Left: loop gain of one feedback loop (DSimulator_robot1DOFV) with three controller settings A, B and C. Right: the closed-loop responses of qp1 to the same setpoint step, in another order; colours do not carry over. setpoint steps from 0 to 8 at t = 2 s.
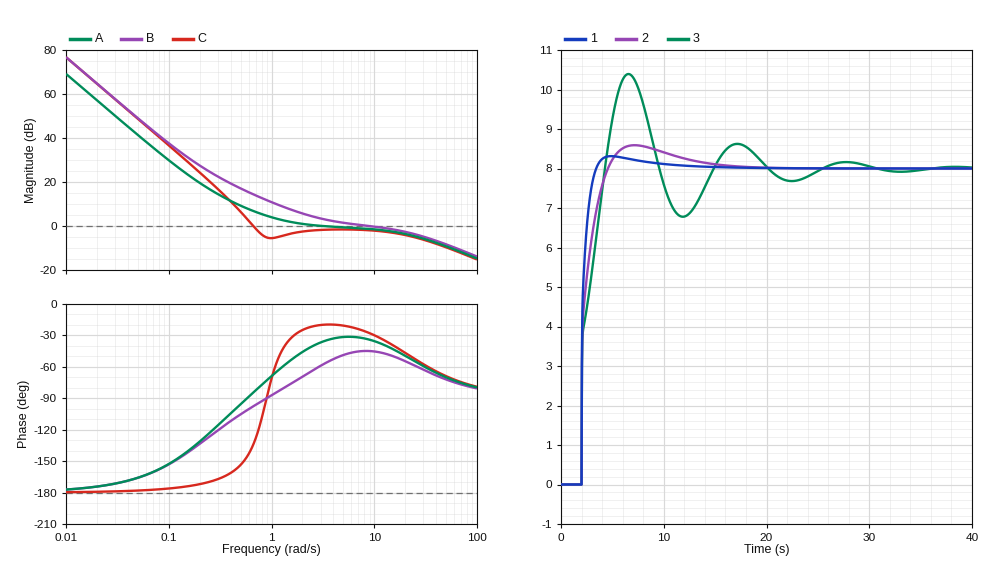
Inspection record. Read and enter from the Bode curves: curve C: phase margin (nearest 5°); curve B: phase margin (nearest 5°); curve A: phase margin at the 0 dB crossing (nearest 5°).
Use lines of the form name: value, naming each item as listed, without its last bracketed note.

curve C: phase margin: 45°
curve B: phase margin: 135°
curve A: phase margin at the 0 dB crossing: 145°
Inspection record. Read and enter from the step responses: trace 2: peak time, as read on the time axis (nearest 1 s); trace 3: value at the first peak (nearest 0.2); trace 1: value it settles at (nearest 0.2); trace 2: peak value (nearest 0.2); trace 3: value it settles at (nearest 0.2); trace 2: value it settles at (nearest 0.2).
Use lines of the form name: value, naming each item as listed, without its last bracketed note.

trace 2: peak time, as read on the time axis: 7 s
trace 3: value at the first peak: 10.4
trace 1: value it settles at: 8.0
trace 2: peak value: 8.6
trace 3: value it settles at: 8.0
trace 2: value it settles at: 8.0
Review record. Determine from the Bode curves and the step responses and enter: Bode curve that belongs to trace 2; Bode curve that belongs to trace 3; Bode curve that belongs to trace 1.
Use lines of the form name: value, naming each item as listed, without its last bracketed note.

Bode curve that belongs to trace 2: A
Bode curve that belongs to trace 3: C
Bode curve that belongs to trace 1: B
